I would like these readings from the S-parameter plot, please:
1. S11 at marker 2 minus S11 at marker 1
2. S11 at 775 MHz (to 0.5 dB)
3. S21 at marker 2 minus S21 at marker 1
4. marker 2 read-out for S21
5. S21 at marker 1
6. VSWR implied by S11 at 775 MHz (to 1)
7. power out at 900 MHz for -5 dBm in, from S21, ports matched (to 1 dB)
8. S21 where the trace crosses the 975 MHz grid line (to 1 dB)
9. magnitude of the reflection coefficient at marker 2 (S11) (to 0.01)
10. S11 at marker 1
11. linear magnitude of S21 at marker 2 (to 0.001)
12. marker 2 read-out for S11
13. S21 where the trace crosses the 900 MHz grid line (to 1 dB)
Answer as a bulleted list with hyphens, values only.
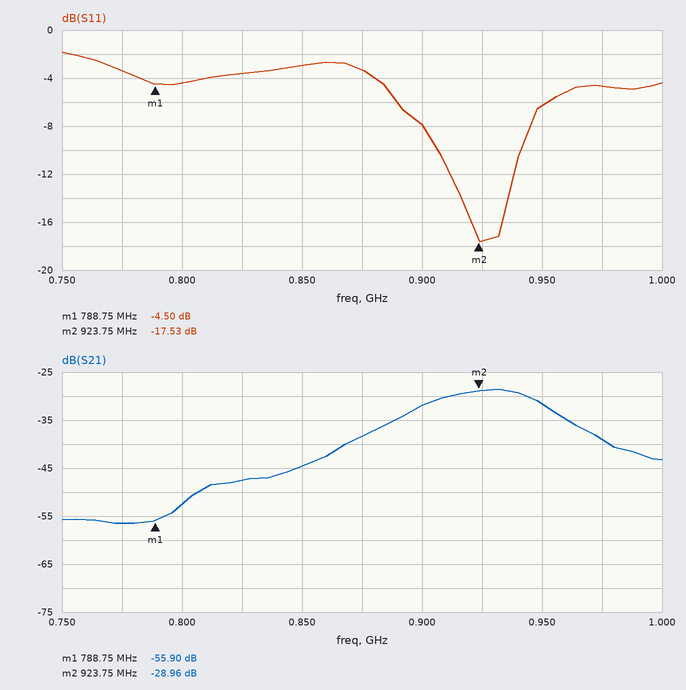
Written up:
- -13.03 dB
- -3.5 dB
- 26.94 dB
- -28.96 dB
- -55.90 dB
- 5
- -37 dBm
- -39 dB
- 0.13
- -4.50 dB
- 0.036
- -17.53 dB
- -32 dB
